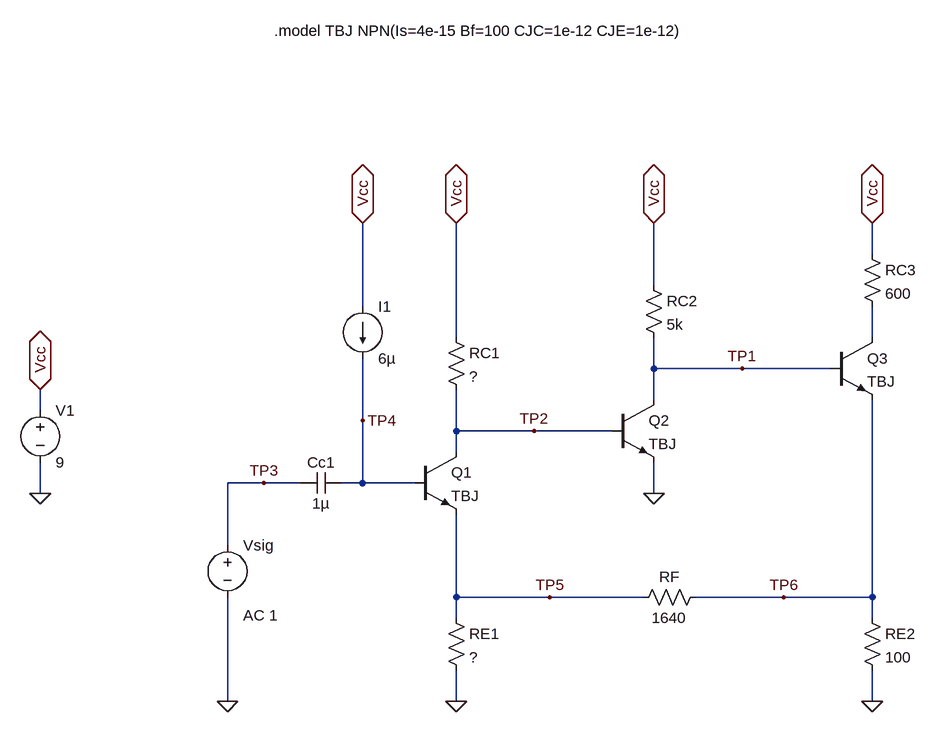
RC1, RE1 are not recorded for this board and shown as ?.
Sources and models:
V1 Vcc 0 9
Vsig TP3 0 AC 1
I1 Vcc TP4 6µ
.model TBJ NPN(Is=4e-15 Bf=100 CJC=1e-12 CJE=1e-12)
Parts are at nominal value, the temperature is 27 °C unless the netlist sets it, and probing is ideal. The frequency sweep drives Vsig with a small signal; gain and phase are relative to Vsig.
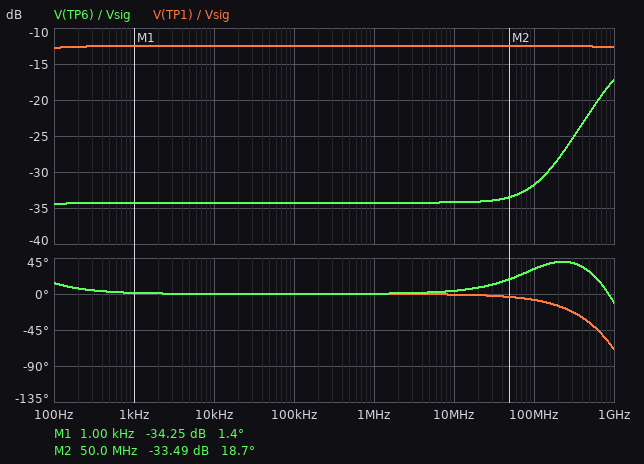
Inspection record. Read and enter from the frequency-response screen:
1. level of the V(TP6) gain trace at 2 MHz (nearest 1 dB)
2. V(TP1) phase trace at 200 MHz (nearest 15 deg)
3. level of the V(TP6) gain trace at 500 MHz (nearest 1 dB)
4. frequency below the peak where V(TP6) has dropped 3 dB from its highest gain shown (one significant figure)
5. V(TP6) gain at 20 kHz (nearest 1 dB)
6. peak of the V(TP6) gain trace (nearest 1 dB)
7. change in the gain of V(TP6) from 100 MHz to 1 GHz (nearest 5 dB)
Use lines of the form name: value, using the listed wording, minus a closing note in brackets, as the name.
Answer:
level of the V(TP6) gain trace at 2 MHz: -34 dB
V(TP1) phase trace at 200 MHz: -15 deg
level of the V(TP6) gain trace at 500 MHz: -22 dB
frequency below the peak where V(TP6) has dropped 3 dB from its highest gain shown: 600 MHz
V(TP6) gain at 20 kHz: -34 dB
peak of the V(TP6) gain trace: -17 dB
change in the gain of V(TP6) from 100 MHz to 1 GHz: 15 dB
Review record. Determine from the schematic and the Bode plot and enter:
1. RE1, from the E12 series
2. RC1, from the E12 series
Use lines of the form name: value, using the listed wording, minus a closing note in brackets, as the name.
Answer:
RE1, from the E12 series: 22 Ω
RC1, from the E12 series: 5.6 kΩ
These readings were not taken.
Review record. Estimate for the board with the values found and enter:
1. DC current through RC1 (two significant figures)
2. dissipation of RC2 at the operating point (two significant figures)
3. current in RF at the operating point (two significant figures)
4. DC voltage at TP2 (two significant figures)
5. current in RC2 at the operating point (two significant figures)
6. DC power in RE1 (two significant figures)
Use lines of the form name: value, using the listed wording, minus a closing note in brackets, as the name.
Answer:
DC current through RC1: 1.5 mA
dissipation of RC2 at the operating point: 16 mW
current in RF at the operating point: 7.6 µA
DC voltage at TP2: 710 mV
current in RC2 at the operating point: 1.8 mA
DC power in RE1: 7.9 µW
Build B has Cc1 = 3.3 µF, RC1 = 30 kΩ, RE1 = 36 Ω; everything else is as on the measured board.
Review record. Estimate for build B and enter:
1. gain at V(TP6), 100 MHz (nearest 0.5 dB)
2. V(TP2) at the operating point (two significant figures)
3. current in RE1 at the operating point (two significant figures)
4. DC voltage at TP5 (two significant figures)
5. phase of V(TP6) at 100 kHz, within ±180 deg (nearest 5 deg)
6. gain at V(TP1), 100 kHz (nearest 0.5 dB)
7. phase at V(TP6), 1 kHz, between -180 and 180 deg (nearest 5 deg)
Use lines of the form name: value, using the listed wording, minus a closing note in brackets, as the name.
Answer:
gain at V(TP6), 100 MHz: -18.0 dB
V(TP2) at the operating point: 160 mV
current in RE1 at the operating point: 1.1 mA
DC voltage at TP5: 39 mV
phase of V(TP6) at 100 kHz, within ±180 deg: -5 deg
gain at V(TP1), 100 kHz: -40.5 dB
phase at V(TP6), 1 kHz, between -180 and 180 deg: 10 deg
